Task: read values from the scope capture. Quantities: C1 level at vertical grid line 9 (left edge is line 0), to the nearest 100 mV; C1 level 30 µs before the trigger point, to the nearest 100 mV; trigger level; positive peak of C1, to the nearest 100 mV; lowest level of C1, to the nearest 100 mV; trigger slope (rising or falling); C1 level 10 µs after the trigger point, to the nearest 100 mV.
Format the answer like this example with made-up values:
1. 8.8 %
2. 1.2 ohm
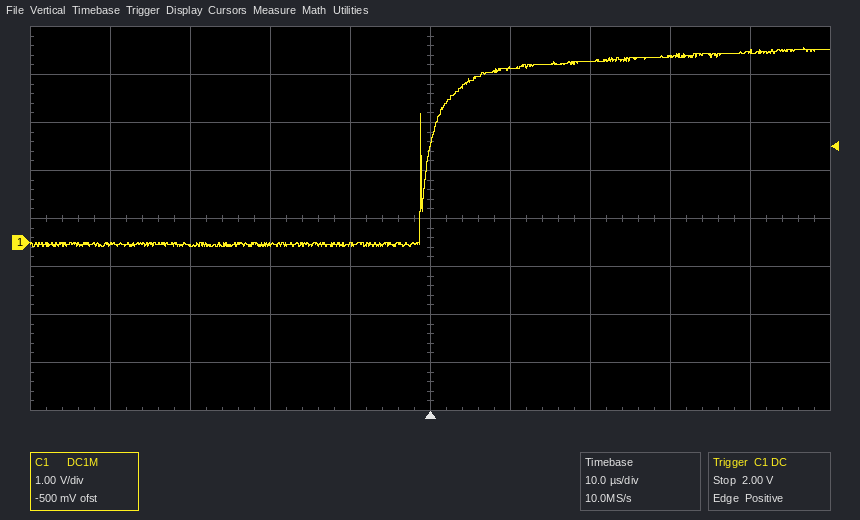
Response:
1. 4.0 V
2. -100 mV
3. 2.00 V
4. 4.1 V
5. -100 mV
6. rising
7. 3.6 V
